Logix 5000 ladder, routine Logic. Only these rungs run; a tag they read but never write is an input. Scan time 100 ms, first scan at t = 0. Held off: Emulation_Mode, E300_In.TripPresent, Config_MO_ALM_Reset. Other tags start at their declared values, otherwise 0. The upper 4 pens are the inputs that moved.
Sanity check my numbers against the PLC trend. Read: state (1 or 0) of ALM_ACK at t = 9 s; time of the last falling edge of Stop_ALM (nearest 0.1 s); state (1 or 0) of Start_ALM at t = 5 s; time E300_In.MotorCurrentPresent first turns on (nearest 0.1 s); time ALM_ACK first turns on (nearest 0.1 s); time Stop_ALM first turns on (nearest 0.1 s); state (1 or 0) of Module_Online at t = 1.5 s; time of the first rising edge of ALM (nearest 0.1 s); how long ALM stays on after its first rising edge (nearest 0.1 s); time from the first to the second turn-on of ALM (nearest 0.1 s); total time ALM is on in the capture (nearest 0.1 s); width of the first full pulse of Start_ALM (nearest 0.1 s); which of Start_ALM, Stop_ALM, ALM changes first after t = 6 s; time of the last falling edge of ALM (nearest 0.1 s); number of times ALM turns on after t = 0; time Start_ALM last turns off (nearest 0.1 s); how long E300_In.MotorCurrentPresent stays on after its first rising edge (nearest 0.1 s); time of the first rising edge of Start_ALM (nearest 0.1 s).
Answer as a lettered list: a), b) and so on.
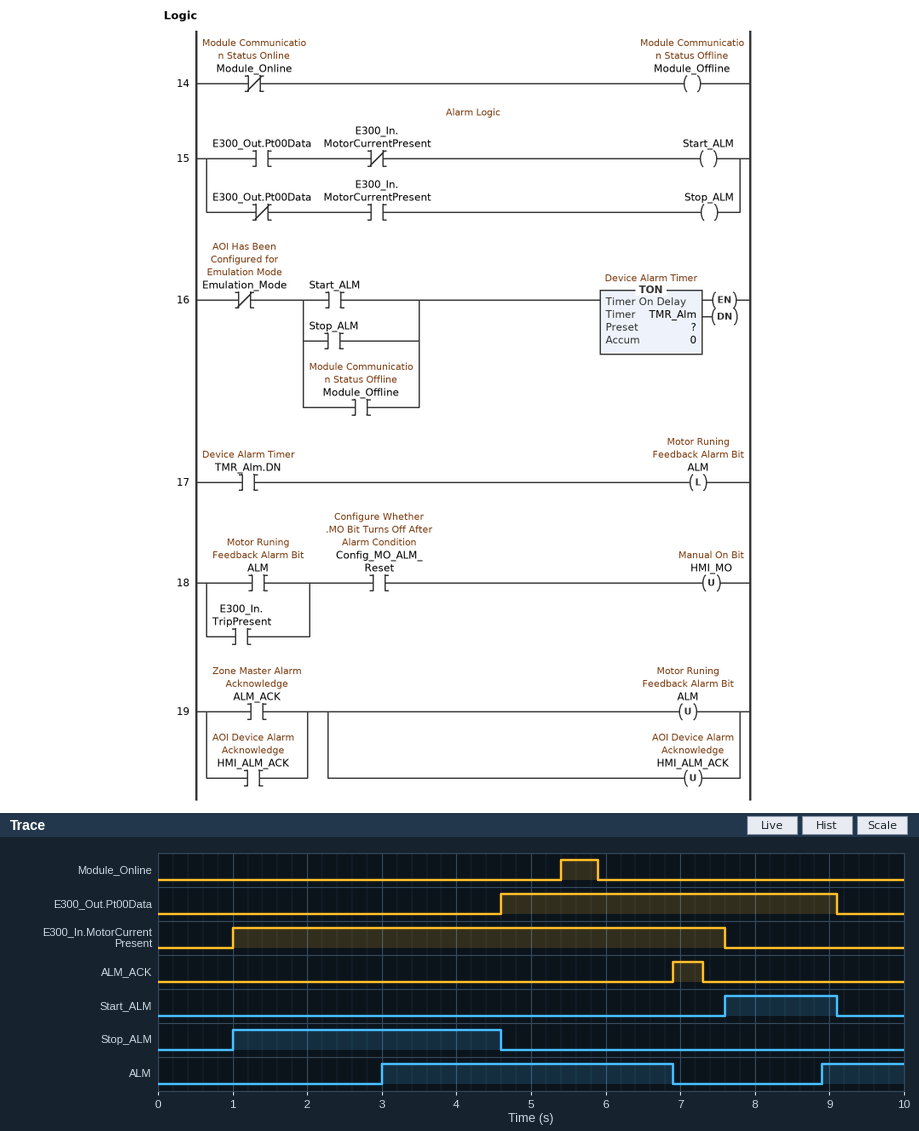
a) 0
b) 4.6 s
c) 0
d) 1.0 s
e) 6.9 s
f) 1.0 s
g) 0
h) 3.0 s
i) 3.9 s
j) 5.9 s
k) 5.0 s
l) 1.5 s
m) ALM
n) 6.9 s
o) 2
p) 9.1 s
q) 6.6 s
r) 7.6 s
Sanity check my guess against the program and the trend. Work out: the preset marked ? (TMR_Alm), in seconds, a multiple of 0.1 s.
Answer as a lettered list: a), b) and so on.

a) 3.0 s
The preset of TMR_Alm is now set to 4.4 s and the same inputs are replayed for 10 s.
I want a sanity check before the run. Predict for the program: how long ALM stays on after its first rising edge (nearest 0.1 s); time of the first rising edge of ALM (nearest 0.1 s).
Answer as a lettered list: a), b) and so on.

a) 2.5 s
b) 4.4 s
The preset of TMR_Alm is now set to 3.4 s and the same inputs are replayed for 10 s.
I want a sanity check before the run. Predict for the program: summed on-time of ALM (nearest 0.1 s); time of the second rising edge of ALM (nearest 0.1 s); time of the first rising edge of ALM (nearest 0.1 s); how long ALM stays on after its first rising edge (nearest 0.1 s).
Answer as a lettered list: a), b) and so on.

a) 4.2 s
b) 9.3 s
c) 3.4 s
d) 3.5 s
